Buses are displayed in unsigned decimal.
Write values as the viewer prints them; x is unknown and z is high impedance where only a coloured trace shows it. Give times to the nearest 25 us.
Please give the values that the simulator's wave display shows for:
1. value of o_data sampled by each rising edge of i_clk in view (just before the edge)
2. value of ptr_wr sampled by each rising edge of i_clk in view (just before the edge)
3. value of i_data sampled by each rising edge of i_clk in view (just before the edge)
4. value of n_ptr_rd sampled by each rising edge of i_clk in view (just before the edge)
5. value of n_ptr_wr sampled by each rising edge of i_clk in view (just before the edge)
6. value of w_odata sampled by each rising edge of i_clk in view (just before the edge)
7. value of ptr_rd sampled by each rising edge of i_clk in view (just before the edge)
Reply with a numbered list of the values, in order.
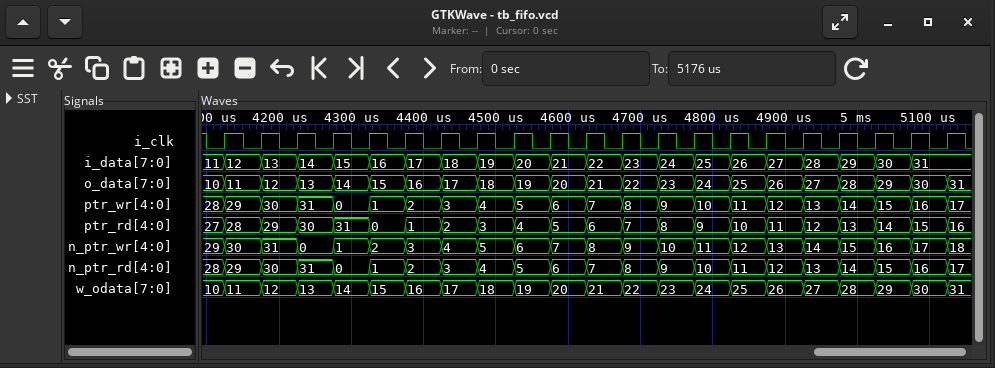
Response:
1. 10, 11, 12, 13, 14, 15, 16, 17, 18, 19, 20, 21, 22, 23, 24, 25, 26, 27, 28, 29, 30
2. 28, 29, 30, 31, 0, 1, 2, 3, 4, 5, 6, 7, 8, 9, 10, 11, 12, 13, 14, 15, 16
3. 11, 12, 13, 14, 15, 16, 17, 18, 19, 20, 21, 22, 23, 24, 25, 26, 27, 28, 29, 30, 31
4. 28, 29, 30, 31, 0, 1, 2, 3, 4, 5, 6, 7, 8, 9, 10, 11, 12, 13, 14, 15, 16
5. 29, 30, 31, 0, 1, 2, 3, 4, 5, 6, 7, 8, 9, 10, 11, 12, 13, 14, 15, 16, 17
6. 10, 11, 12, 13, 14, 15, 16, 17, 18, 19, 20, 21, 22, 23, 24, 25, 26, 27, 28, 29, 30
7. 27, 28, 29, 30, 31, 0, 1, 2, 3, 4, 5, 6, 7, 8, 9, 10, 11, 12, 13, 14, 15
